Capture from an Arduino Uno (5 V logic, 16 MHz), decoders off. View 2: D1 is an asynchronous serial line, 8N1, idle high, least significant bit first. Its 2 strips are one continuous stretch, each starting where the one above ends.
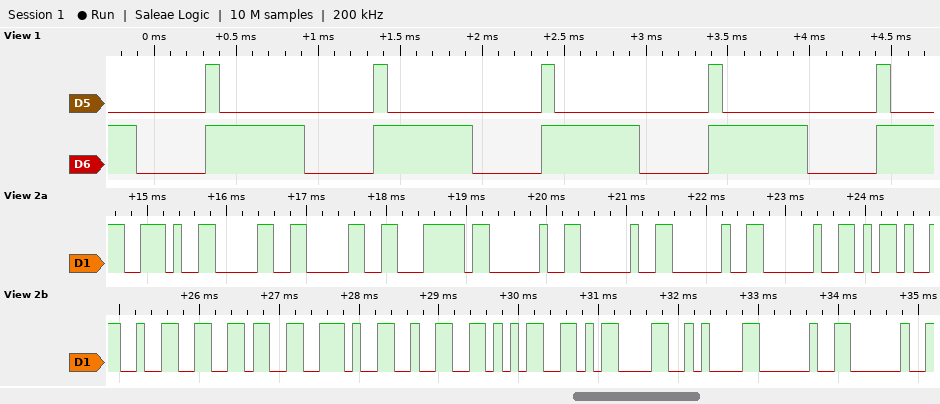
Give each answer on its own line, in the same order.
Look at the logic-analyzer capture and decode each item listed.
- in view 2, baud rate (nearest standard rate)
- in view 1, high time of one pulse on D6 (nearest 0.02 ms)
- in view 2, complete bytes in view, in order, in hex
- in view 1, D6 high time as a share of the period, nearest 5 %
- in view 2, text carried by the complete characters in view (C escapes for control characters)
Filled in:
9600 baud
0.60 ms
0x2E 0x30 0x30 0x7C 0x20 0x20 0x20 0x20 0x2D 0x32 0x36 0x2E 0x32 0x35 0x0D 0x0A 0x20 0x20
60 %
".00|    -26.25\r\n  "
